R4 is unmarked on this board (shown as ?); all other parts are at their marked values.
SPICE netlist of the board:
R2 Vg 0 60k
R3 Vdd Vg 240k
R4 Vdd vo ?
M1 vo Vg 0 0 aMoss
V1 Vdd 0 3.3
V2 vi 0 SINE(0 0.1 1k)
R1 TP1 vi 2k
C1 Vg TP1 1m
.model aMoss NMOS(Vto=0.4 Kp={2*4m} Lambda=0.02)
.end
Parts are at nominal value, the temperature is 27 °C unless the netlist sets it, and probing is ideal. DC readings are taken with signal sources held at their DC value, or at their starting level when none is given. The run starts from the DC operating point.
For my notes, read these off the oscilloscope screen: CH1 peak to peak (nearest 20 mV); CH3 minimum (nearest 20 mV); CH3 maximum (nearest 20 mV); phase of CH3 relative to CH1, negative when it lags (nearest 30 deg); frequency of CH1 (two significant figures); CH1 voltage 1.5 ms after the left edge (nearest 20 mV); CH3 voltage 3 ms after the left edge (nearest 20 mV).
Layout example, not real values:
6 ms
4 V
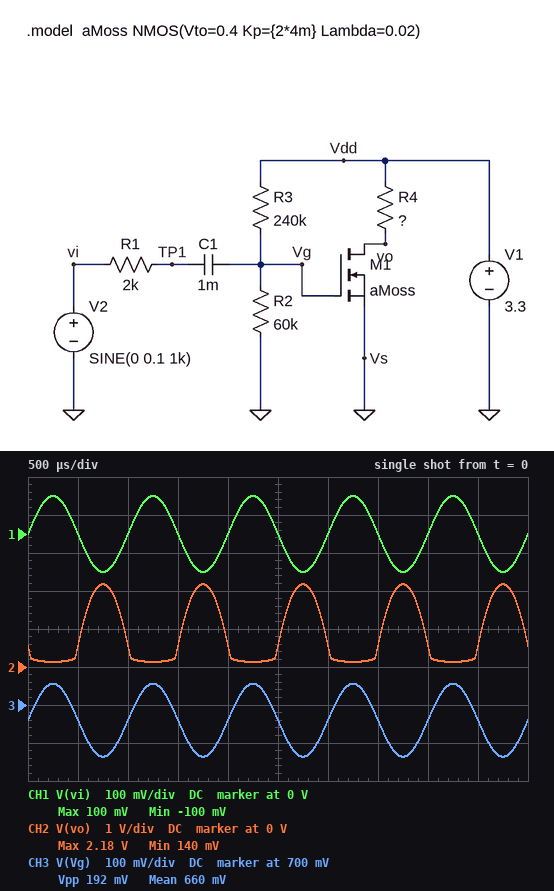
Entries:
200 mV
560 mV
760 mV
0 deg
1.0 kHz
0 V
660 mV
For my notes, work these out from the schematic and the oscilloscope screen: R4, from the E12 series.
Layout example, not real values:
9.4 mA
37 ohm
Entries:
10 kΩ
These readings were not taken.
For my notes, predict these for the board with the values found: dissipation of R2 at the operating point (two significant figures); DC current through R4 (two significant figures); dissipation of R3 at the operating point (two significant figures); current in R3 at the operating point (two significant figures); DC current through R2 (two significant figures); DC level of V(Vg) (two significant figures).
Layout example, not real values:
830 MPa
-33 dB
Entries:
7.3 µW
270 µA
29 µW
11 µA
11 µA
660 mV
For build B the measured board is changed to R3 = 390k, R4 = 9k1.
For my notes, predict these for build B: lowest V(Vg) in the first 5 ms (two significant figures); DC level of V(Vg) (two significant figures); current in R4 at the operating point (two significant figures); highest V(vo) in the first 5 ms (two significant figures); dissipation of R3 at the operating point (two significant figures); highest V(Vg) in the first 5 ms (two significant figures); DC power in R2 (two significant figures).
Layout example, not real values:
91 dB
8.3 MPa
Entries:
340 mV
440 mV
6.8 µA
3.3 V
21 µW
540 mV
3.2 µW
